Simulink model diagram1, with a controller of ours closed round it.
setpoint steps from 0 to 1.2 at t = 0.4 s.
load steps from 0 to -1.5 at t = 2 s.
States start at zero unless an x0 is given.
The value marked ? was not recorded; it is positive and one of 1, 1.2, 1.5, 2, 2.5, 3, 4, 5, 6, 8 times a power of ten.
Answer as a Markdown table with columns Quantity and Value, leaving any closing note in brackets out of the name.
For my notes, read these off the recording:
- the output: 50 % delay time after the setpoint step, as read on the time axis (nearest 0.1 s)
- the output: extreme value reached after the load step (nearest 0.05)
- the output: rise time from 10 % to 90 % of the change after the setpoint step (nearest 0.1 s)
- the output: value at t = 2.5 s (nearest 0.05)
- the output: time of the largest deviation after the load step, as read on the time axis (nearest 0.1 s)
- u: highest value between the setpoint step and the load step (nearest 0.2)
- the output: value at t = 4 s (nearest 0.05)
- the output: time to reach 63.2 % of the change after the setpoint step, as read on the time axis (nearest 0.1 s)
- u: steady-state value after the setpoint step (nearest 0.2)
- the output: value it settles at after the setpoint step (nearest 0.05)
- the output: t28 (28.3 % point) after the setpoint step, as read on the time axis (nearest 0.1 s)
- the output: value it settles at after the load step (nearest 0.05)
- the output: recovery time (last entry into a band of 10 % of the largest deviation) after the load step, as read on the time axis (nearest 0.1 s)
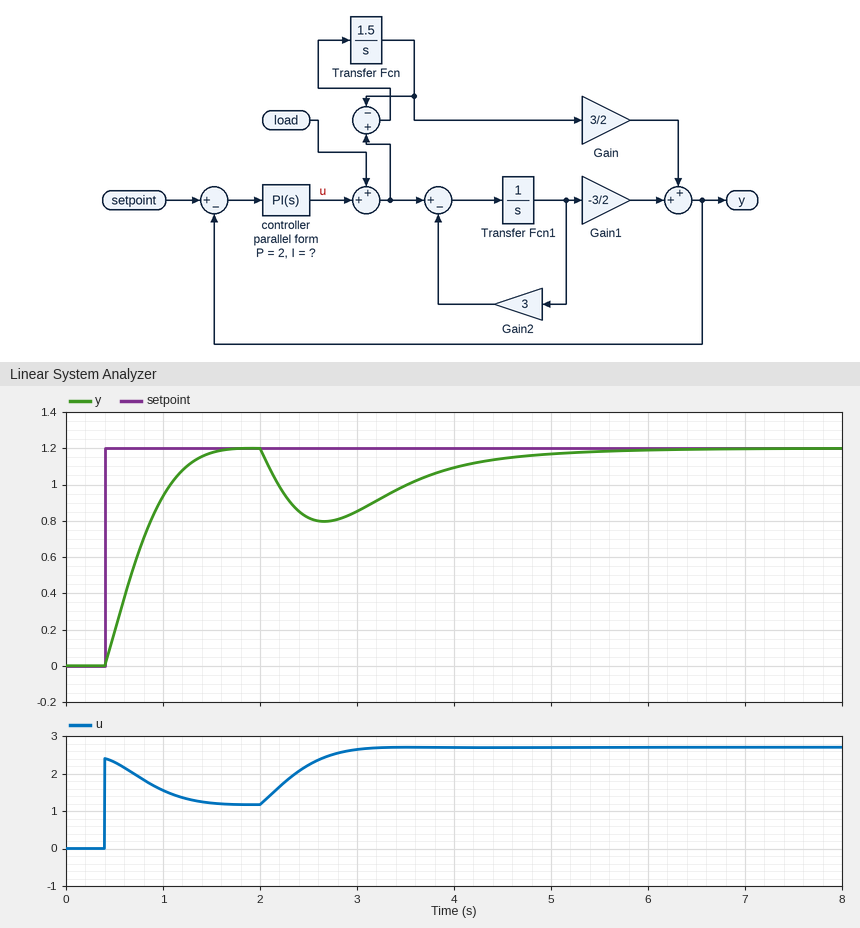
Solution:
| Quantity | Value |
|---|---|
| the output: 50 % delay time after the setpoint step, as read on the time axis | 0.7 s |
| the output: extreme value reached after the load step | 0.80 |
| the output: rise time from 10 % to 90 % of the change after the setpoint step | 0.7 s |
| the output: value at t = 2.5 s | 0.80 |
| the output: time of the largest deviation after the load step, as read on the time axis | 2.7 s |
| u: highest value between the setpoint step and the load step | 2.4 |
| the output: value at t = 4 s | 1.10 |
| the output: time to reach 63.2 % of the change after the setpoint step, as read on the time axis | 0.8 s |
| u: steady-state value after the setpoint step | 1.2 |
| the output: value it settles at after the setpoint step | 1.20 |
| the output: t28 (28.3 % point) after the setpoint step, as read on the time axis | 0.6 s |
| the output: value it settles at after the load step | 1.20 |
| the output: recovery time (last entry into a band of 10 % of the largest deviation) after the load step, as read on the time axis | 4.8 s |
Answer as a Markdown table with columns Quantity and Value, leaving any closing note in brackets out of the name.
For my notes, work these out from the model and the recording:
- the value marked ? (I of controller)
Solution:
| Quantity | Value |
|---|---|
| the value marked ? | 2.5 |
